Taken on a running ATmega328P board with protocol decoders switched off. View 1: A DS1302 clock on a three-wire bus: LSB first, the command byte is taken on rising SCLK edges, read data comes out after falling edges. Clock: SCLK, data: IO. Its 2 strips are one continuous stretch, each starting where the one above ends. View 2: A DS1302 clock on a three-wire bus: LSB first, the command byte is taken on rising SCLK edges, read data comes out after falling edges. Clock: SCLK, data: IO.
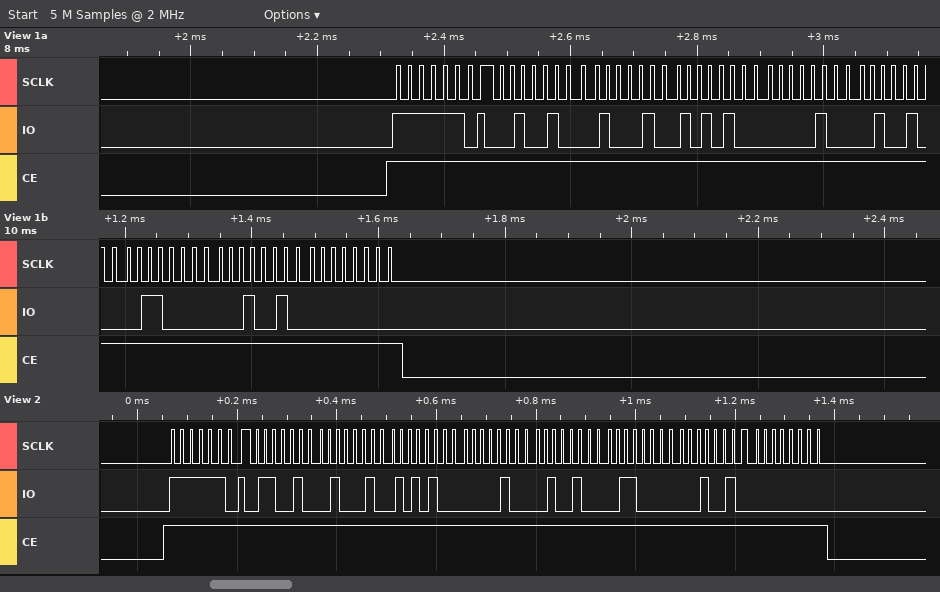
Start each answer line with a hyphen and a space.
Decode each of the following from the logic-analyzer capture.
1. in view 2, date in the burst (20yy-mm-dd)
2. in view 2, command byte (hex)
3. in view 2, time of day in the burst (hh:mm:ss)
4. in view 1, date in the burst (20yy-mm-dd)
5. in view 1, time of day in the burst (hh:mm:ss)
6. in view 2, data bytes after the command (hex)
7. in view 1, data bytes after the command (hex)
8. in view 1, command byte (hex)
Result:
- 2024-12-10
- 0xBF
- 15:22:26
- 2024-12-10
- 15:22:24
- 26 22 15 10 12 06 24 00
- 24 22 15 10 12 06 24 00
- 0xBF
